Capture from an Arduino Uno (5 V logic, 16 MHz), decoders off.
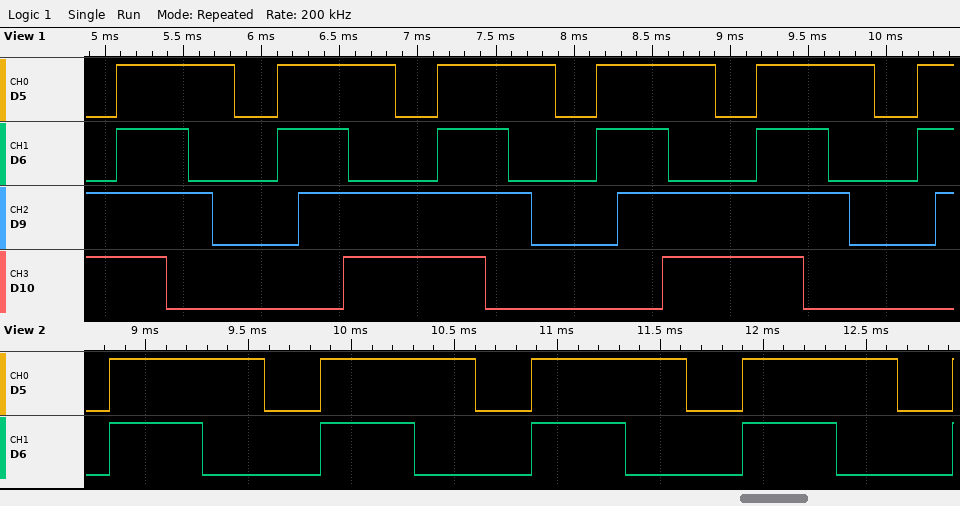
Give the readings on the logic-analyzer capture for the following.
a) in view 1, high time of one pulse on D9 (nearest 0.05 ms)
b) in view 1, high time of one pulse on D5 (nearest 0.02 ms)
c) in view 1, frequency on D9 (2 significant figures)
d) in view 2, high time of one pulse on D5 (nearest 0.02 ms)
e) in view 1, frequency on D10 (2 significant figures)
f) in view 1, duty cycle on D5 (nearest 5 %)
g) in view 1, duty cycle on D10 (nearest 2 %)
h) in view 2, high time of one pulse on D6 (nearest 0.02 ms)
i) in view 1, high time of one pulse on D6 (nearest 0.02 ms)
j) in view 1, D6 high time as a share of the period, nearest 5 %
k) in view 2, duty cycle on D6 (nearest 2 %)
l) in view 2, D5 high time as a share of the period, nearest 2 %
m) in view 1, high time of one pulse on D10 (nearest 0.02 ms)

1.50 ms
0.76 ms
490 Hz
0.76 ms
490 Hz
75 %
44 %
0.46 ms
0.46 ms
45 %
44 %
74 %
0.90 ms
